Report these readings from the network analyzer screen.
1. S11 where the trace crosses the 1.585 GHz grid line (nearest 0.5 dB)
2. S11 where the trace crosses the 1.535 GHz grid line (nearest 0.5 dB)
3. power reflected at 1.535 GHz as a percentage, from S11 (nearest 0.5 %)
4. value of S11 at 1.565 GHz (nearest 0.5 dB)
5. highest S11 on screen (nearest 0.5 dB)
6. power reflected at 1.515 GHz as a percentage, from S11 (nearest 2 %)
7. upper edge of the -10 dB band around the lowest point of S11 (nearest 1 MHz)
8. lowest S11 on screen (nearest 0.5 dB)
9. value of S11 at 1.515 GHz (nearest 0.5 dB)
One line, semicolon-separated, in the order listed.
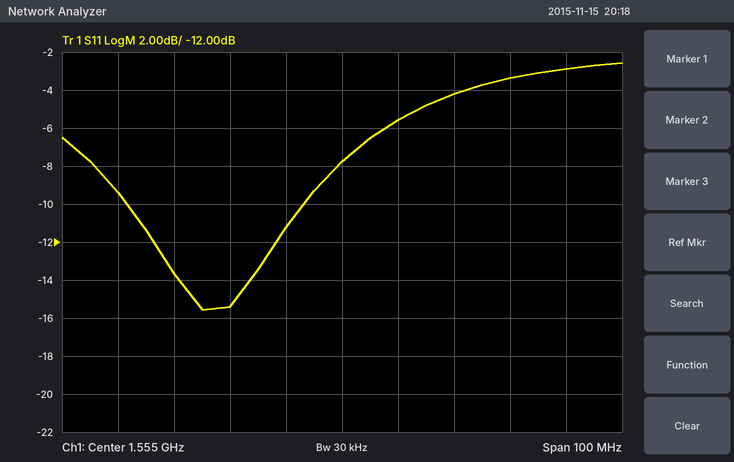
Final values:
-3.5 dB; -15.5 dB; 3.0 %; -5.5 dB; -2.5 dB; 12 %; 1.548 GHz; -15.5 dB; -9.5 dB
